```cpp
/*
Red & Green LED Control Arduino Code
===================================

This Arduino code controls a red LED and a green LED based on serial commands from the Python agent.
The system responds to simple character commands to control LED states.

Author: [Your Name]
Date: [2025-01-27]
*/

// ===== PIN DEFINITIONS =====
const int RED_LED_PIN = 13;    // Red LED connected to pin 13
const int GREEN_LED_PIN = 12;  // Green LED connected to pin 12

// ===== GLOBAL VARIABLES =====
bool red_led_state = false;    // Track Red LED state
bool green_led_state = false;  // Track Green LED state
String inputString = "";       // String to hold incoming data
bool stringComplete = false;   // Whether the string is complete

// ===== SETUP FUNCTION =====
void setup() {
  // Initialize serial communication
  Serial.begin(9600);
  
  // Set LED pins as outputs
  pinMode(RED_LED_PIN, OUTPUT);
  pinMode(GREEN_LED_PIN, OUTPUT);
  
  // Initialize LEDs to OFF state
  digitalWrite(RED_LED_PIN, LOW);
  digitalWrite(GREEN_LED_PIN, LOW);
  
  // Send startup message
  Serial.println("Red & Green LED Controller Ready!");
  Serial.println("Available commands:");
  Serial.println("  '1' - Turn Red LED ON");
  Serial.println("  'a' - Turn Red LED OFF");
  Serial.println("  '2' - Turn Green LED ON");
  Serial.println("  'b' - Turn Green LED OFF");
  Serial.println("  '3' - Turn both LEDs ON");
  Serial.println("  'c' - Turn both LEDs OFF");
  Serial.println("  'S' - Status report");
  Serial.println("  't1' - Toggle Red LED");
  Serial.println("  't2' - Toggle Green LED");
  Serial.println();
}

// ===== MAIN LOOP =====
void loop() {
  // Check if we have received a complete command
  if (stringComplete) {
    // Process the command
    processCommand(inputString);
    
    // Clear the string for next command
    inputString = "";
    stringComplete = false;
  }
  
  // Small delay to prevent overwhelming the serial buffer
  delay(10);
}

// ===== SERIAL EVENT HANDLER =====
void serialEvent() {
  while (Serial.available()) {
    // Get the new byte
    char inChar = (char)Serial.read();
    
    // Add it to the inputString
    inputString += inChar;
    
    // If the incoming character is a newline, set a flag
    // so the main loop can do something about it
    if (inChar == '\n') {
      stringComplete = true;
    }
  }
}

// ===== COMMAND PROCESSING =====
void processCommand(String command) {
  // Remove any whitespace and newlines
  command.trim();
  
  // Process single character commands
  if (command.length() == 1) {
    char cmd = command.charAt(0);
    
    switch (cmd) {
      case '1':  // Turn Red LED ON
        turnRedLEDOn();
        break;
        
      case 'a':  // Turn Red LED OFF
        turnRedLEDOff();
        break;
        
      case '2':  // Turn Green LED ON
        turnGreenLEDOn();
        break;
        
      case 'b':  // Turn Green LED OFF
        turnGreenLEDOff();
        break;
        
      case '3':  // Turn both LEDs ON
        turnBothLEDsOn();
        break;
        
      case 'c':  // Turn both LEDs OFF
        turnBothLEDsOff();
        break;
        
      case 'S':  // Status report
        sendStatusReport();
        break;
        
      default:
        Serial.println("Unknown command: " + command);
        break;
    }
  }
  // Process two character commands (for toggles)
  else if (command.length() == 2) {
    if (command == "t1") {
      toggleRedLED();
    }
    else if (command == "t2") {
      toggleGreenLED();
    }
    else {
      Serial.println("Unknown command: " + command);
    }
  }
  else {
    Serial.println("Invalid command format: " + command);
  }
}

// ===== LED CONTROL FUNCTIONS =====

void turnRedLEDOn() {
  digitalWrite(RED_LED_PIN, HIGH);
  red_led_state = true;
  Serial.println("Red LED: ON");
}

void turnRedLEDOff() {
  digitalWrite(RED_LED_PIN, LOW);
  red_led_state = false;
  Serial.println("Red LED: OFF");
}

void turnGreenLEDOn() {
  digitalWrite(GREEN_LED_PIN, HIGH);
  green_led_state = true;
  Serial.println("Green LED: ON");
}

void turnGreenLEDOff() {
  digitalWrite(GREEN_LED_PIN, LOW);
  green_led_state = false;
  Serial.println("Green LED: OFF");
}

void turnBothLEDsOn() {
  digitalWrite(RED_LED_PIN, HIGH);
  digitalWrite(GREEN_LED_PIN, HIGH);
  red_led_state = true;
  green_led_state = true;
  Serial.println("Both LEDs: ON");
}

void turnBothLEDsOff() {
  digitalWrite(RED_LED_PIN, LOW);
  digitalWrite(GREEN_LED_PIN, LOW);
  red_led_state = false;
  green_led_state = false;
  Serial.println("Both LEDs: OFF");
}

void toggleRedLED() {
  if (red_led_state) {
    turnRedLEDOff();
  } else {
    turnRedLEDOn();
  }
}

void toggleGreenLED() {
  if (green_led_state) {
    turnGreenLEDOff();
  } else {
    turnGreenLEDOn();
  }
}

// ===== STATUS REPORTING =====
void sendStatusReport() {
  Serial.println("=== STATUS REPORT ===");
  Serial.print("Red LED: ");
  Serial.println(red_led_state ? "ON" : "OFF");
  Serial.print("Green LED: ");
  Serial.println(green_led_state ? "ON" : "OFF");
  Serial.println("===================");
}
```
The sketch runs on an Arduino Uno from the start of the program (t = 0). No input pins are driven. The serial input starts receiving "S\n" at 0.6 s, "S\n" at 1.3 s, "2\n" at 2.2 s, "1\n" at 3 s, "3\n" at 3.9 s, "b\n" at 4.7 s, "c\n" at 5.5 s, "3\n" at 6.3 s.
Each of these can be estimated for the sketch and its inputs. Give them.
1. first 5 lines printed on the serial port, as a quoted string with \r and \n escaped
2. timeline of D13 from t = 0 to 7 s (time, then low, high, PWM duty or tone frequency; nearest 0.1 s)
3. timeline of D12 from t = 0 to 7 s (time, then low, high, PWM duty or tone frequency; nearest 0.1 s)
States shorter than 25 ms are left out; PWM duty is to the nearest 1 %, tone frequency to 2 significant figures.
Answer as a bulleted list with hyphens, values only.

- "Red & Green LED Controller Ready!\r\nAvailable commands:\r\n  '1' - Turn Red LED ON\r\n  'a' - Turn Red LED OFF\r\n  '2' - Turn Green LED ON\r\n"
- 0 s low; 3 s high; 5.5 s low; 6.3 s high
- 0 s low; 2.2 s high; 4.7 s low; 6.3 s high
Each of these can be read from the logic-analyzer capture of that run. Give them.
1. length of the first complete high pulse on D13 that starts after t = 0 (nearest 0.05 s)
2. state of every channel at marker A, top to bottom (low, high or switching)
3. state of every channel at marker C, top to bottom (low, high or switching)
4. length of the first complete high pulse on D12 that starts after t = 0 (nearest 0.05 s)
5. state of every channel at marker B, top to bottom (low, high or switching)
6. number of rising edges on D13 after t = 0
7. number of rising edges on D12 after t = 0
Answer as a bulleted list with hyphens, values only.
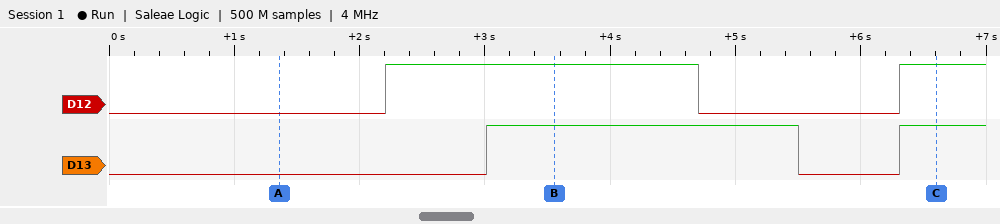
- 2.50 s
- D12 low, D13 low
- D12 high, D13 high
- 2.50 s
- D12 high, D13 high
- 2
- 2
